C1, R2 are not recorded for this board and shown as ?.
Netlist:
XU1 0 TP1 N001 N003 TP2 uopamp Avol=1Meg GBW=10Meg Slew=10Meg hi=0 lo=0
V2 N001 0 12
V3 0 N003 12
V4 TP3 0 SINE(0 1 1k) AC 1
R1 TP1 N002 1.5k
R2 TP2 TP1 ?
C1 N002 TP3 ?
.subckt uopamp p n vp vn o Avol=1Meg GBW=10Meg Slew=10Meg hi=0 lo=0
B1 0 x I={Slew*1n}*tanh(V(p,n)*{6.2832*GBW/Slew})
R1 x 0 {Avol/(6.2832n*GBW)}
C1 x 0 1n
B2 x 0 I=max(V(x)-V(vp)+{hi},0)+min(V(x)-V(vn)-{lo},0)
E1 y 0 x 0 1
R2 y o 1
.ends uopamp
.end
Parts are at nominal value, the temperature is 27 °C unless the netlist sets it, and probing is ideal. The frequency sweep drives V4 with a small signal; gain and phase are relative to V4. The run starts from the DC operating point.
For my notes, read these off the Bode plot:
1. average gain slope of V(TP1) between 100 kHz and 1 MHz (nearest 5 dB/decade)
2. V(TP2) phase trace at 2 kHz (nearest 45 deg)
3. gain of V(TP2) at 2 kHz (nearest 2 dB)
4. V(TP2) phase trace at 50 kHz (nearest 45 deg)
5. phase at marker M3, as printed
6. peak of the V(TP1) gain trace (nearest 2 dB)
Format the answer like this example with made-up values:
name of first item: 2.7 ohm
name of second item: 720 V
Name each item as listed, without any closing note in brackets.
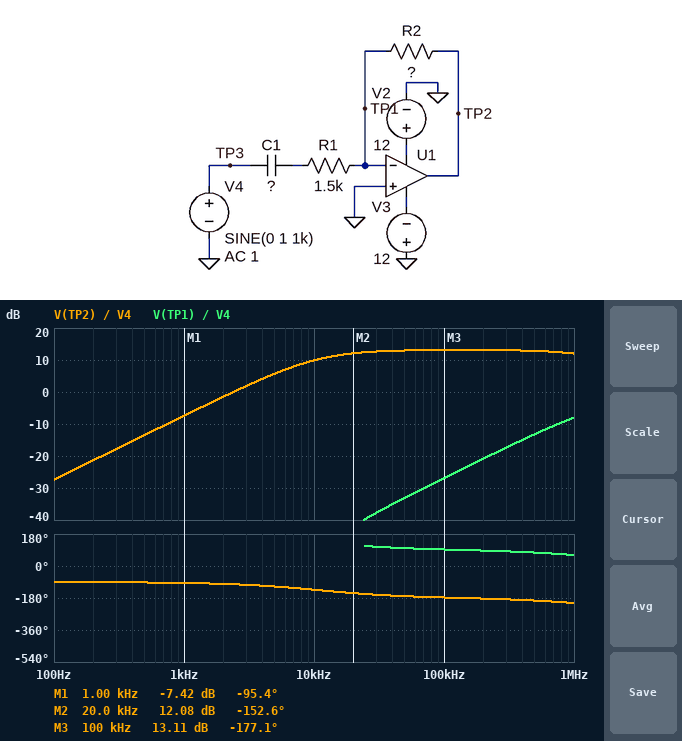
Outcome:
average gain slope of V(TP1) between 100 kHz and 1 MHz: 20 dB/decade
V(TP2) phase trace at 2 kHz: -90 deg
gain of V(TP2) at 2 kHz: -2 dB
V(TP2) phase trace at 50 kHz: -180 deg
phase at marker M3, as printed: -177.1 deg
peak of the V(TP1) gain trace: -8 dB
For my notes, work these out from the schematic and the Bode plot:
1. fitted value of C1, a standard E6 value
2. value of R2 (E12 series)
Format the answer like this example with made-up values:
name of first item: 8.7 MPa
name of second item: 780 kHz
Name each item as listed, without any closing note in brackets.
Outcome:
fitted value of C1, a standard E6 value: 10 nF
value of R2: 6.8 kΩ
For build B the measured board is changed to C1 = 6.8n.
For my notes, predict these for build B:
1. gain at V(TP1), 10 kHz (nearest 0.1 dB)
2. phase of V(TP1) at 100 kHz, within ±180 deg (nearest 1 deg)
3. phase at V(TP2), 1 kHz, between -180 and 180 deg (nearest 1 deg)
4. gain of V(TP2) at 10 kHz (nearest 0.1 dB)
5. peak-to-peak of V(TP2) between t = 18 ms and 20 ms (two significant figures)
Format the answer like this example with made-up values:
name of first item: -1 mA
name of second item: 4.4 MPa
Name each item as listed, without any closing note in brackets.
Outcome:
gain at V(TP1), 10 kHz: -52.2 dB
phase of V(TP1) at 100 kHz, within ±180 deg: 96 deg
phase at V(TP2), 1 kHz, between -180 and 180 deg: -94 deg
gain of V(TP2) at 10 kHz: 7.8 dB
peak-to-peak of V(TP2) between t = 18 ms and 20 ms: 580 mV
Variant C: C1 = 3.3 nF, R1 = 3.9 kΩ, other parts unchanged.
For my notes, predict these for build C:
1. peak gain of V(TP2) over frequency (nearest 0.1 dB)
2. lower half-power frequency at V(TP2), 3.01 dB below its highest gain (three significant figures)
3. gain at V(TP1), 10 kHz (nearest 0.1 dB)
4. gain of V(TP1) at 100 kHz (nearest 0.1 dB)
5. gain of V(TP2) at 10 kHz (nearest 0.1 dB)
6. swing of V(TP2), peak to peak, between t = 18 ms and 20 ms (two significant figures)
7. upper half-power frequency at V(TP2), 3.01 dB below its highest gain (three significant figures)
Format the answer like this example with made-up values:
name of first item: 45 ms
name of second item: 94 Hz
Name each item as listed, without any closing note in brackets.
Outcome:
peak gain of V(TP2) over frequency: 4.8 dB
lower half-power frequency at V(TP2), 3.01 dB below its highest gain: 12.3 kHz
gain at V(TP1), 10 kHz: -59.2 dB
gain of V(TP1) at 100 kHz: -35.2 dB
gain of V(TP2) at 10 kHz: 0.8 dB
swing of V(TP2), peak to peak, between t = 18 ms and 20 ms: 280 mV
upper half-power frequency at V(TP2), 3.01 dB below its highest gain: 3.66 MHz
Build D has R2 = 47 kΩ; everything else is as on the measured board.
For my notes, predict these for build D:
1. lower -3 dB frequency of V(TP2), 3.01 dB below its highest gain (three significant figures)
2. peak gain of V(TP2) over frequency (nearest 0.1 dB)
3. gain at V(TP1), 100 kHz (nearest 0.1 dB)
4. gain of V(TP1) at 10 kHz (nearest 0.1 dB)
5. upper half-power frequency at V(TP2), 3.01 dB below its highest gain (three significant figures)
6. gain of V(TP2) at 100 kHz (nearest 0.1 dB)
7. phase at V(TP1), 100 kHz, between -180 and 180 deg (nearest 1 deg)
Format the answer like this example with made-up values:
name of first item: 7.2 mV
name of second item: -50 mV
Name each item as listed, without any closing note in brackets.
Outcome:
lower -3 dB frequency of V(TP2), 3.01 dB below its highest gain: 10.3 kHz
peak gain of V(TP2) over frequency: 29.9 dB
gain at V(TP1), 100 kHz: -10.3 dB
gain of V(TP1) at 10 kHz: -33.2 dB
upper half-power frequency at V(TP2), 3.01 dB below its highest gain: 320 kHz
gain of V(TP2) at 100 kHz: 29.7 dB
phase at V(TP1), 100 kHz, between -180 and 180 deg: 78 deg
